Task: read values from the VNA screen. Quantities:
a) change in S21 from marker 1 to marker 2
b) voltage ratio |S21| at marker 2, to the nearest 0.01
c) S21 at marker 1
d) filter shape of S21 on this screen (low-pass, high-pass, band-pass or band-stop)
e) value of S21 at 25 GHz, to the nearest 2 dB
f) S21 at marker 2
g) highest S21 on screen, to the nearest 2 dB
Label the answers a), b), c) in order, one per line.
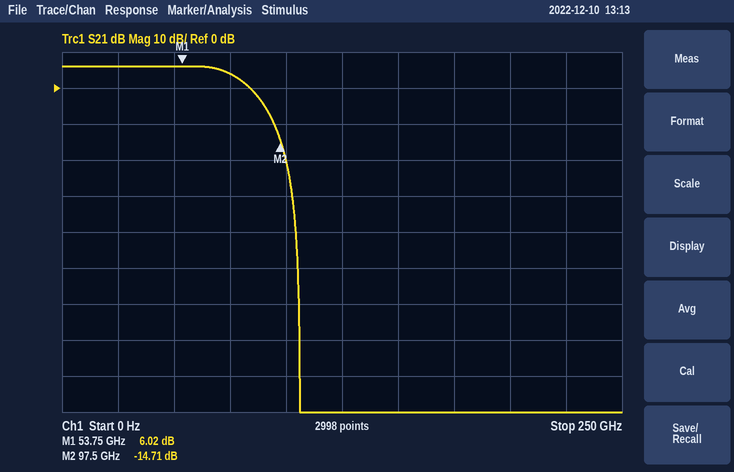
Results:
a) -20.73 dB
b) 0.18
c) 6.02 dB
d) low-pass
e) 6 dB
f) -14.71 dB
g) 6 dB
